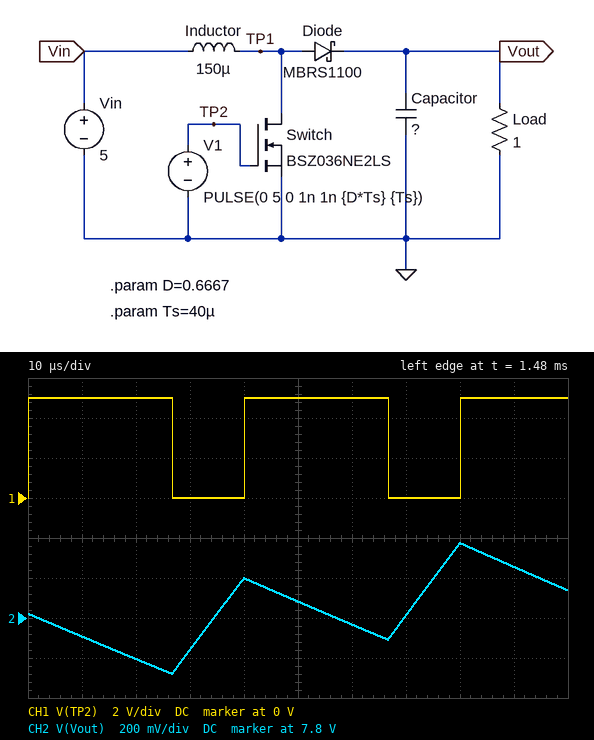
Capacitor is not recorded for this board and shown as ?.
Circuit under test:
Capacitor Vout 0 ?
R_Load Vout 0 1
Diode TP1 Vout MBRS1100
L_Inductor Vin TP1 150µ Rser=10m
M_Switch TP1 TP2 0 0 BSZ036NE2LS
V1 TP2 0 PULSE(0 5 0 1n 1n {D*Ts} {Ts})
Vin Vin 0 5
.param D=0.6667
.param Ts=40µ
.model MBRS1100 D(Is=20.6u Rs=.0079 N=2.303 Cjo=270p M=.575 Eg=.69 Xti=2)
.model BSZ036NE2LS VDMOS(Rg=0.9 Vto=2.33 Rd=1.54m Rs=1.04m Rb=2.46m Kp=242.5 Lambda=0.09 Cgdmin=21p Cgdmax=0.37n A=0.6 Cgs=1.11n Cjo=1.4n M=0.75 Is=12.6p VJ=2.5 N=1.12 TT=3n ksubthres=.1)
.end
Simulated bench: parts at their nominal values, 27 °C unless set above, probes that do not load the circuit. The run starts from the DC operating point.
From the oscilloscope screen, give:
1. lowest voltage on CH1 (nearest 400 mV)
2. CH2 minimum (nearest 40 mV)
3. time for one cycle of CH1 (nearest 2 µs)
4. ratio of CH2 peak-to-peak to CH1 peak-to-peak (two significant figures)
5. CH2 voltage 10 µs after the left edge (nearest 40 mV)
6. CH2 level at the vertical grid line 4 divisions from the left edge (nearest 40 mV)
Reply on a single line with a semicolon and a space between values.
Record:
0 V; 7.52 V; 40 µs; 0.13; 7.72 V; 8.00 V
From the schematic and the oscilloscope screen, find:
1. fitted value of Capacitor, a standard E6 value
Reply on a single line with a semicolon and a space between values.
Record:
680 µF
